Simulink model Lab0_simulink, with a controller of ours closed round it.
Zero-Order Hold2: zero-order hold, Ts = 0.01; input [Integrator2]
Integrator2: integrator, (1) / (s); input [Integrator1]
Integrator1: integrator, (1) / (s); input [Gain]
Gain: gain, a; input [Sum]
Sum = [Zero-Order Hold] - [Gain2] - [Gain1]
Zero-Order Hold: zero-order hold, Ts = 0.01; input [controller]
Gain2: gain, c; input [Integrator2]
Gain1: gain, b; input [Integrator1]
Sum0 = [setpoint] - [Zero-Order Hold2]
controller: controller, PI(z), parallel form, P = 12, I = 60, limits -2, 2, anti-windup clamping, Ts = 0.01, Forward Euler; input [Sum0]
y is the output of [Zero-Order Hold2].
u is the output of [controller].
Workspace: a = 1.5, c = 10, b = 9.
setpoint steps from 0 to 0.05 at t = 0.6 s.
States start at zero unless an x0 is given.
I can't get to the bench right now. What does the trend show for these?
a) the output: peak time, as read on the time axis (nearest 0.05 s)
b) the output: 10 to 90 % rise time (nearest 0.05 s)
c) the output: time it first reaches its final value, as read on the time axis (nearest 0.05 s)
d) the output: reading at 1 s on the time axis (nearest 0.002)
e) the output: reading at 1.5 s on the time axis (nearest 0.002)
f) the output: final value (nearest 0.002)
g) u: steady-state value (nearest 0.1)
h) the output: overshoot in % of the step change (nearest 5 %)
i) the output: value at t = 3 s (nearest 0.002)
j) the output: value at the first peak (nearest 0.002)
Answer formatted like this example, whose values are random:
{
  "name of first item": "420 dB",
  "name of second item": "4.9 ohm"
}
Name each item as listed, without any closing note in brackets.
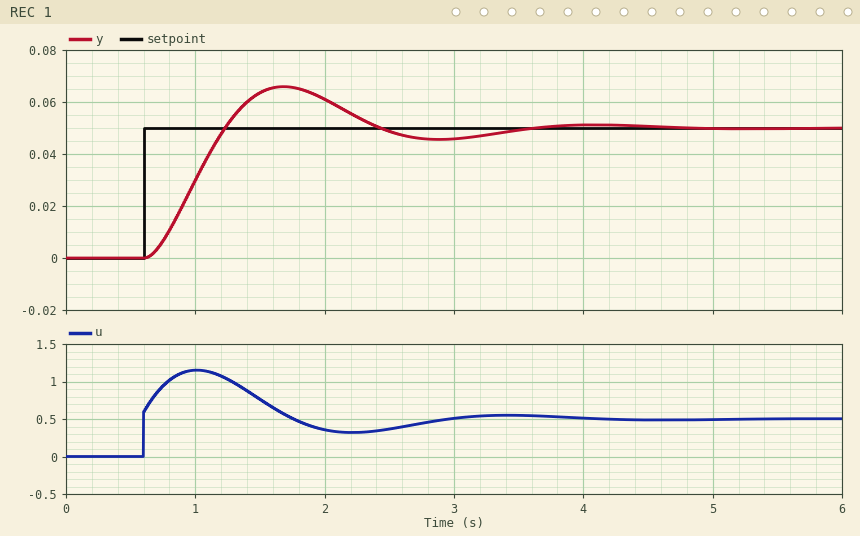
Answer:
{
  "the output: peak time, as read on the time axis": "1.70 s",
  "the output: 10 to 90 % rise time": "0.45 s",
  "the output: time it first reaches its final value, as read on the time axis": "1.25 s",
  "the output: reading at 1 s on the time axis": "0.030",
  "the output: reading at 1.5 s on the time axis": "0.064",
  "the output: final value": "0.050",
  "u: steady-state value": "0.5",
  "the output: overshoot in % of the step change": "30 %",
  "the output: value at t = 3 s": "0.046",
  "the output: value at the first peak": "0.066"
}
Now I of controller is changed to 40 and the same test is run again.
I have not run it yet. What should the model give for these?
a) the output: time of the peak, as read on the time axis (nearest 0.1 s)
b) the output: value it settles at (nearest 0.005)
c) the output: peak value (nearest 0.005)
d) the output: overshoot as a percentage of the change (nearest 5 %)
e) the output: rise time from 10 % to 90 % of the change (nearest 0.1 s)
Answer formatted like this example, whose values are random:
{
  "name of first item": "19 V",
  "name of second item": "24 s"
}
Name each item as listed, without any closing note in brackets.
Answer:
{
  "the output: time of the peak, as read on the time axis": "1.9 s",
  "the output: value it settles at": "0.050",
  "the output: peak value": "0.060",
  "the output: overshoot as a percentage of the change": "20 %",
  "the output: rise time from 10 % to 90 % of the change": "0.6 s"
}
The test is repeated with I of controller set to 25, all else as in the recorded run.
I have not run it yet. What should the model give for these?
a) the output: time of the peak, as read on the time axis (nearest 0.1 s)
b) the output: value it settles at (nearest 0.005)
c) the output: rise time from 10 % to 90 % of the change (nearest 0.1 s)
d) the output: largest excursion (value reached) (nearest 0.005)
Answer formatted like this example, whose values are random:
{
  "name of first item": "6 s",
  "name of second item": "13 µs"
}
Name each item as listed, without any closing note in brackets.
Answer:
{
  "the output: time of the peak, as read on the time axis": "2.3 s",
  "the output: value it settles at": "0.050",
  "the output: rise time from 10 % to 90 % of the change": "0.8 s",
  "the output: largest excursion (value reached)": "0.055"
}
